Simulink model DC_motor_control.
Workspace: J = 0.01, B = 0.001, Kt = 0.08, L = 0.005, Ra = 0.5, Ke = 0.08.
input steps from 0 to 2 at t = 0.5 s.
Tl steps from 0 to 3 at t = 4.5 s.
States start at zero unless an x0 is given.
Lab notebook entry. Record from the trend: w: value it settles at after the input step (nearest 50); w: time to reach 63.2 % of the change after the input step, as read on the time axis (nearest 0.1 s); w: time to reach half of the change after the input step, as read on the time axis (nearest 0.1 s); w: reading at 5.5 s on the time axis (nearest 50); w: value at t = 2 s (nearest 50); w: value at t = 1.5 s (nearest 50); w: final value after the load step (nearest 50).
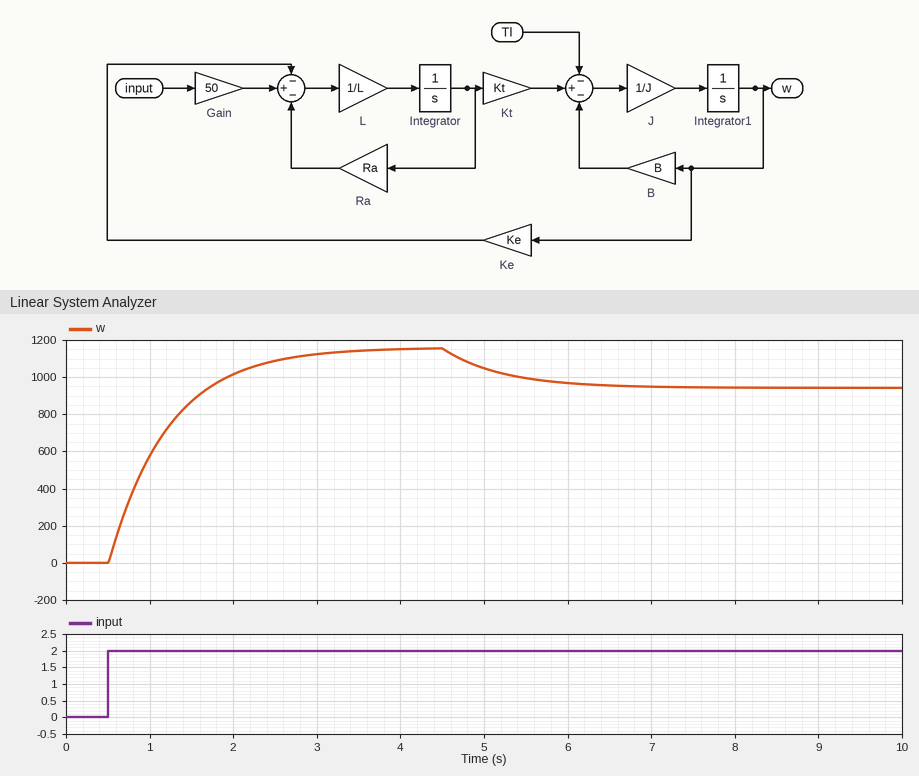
1150
1.2 s
1.0 s
1000
1000
850
950
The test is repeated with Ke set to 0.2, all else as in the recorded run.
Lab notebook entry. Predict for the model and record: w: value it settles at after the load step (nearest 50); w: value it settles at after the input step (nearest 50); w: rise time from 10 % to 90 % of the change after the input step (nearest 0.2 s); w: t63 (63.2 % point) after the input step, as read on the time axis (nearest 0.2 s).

400
500
0.6 s
0.8 s
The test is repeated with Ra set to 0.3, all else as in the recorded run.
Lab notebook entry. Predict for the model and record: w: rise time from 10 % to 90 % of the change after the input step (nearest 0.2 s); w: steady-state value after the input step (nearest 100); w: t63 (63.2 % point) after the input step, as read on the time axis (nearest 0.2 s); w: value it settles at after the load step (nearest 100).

1.0 s
1200
1.0 s
1100
